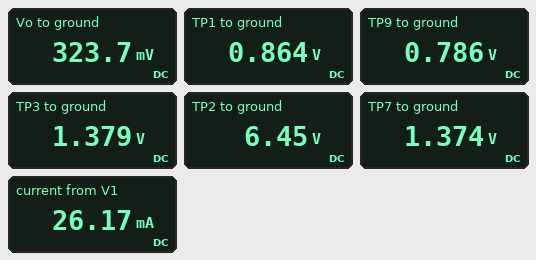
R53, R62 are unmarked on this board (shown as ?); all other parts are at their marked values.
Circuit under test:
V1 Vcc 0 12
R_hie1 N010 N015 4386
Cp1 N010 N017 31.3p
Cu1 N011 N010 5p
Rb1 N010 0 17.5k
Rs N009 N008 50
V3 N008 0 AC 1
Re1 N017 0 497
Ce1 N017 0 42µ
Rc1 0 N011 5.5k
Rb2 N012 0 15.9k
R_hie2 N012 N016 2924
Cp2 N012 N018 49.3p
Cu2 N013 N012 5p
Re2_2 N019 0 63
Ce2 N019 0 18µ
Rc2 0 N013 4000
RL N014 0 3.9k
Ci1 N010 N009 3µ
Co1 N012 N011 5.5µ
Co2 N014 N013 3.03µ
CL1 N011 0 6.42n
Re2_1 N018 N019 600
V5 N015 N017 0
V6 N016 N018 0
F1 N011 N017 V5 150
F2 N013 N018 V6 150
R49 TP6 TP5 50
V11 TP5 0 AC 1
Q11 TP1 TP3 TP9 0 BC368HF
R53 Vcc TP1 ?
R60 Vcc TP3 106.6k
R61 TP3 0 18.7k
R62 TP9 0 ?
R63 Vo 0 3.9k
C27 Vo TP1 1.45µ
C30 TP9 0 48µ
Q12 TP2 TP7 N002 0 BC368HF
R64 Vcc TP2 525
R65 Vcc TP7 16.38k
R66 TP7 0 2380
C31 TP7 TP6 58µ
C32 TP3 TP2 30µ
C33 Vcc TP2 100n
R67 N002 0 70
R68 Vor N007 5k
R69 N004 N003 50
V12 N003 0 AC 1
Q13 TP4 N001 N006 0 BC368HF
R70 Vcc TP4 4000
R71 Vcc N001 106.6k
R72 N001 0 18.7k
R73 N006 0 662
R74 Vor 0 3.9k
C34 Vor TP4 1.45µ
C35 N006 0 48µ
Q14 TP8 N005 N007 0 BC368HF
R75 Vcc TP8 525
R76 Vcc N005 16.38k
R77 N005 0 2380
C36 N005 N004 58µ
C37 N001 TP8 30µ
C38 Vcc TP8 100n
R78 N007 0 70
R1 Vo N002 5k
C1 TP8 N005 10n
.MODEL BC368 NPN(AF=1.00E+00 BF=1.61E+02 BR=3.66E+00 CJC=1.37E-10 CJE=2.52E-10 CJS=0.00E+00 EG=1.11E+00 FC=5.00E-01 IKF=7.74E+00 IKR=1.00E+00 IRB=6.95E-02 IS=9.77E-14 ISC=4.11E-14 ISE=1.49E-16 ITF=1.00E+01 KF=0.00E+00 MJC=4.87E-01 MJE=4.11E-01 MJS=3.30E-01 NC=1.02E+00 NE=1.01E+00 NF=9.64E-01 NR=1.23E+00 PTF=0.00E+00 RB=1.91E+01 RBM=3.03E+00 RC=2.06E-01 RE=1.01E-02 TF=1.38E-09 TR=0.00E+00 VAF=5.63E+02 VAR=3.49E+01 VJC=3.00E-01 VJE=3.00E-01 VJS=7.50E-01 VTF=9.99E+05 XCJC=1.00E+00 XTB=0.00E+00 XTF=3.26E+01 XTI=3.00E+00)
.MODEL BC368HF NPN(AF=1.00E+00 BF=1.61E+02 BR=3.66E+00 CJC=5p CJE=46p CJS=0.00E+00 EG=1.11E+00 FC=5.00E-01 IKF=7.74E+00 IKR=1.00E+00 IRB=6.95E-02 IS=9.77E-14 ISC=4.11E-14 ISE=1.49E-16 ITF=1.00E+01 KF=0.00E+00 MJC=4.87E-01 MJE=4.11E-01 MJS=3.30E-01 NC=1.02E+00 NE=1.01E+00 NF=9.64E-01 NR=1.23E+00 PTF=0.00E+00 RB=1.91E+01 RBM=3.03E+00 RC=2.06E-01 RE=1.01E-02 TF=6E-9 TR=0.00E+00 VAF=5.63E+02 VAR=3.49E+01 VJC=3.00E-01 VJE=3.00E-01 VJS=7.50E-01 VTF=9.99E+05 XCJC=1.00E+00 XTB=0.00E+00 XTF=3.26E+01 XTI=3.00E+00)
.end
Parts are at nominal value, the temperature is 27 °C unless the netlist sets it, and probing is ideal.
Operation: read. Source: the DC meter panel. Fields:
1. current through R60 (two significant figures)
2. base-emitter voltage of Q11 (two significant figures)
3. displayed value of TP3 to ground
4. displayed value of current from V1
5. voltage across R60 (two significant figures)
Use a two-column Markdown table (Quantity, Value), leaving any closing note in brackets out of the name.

| Quantity | Value |
|---|---|
| current through R60 | 100 µA |
| base-emitter voltage of Q11 | 590 mV |
| displayed value of TP3 to ground | 1.379 V |
| displayed value of current from V1 | 26.17 mA |
| voltage across R60 | 11 V |
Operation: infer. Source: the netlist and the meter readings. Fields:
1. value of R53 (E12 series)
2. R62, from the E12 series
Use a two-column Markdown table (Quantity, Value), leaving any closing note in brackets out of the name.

| Quantity | Value |
|---|---|
| value of R53 | 5.6 kΩ |
| R62, from the E12 series | 390 Ω |
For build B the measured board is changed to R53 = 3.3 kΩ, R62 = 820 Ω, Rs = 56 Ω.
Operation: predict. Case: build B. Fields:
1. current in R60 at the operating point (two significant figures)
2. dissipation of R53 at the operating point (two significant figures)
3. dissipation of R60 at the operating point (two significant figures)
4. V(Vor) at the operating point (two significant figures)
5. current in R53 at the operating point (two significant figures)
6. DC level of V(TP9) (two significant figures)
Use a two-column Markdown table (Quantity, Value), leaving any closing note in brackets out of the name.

| Quantity | Value |
|---|---|
| current in R60 at the operating point | 97 µA |
| dissipation of R53 at the operating point | 5.5 mW |
| dissipation of R60 at the operating point | 1.0 mW |
| V(Vor) at the operating point | 320 mV |
| current in R53 at the operating point | 1.3 mA |
| DC level of V(TP9) | 1.1 V |
